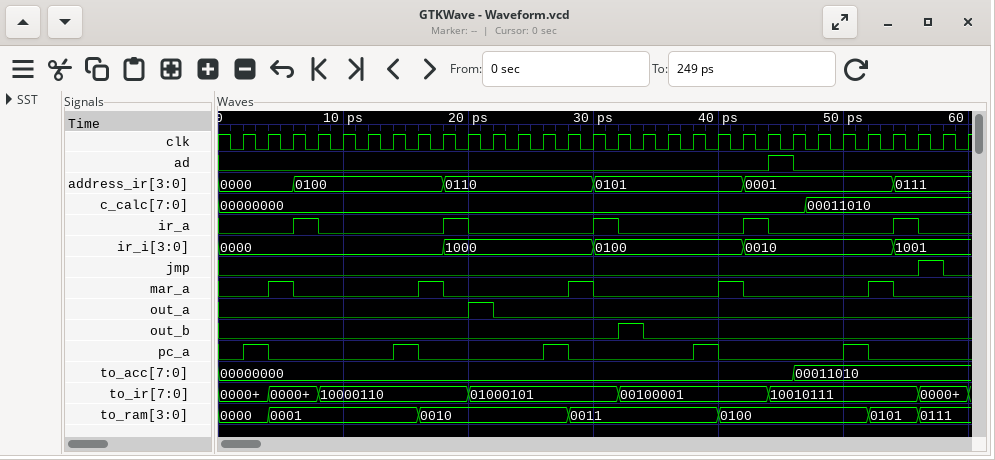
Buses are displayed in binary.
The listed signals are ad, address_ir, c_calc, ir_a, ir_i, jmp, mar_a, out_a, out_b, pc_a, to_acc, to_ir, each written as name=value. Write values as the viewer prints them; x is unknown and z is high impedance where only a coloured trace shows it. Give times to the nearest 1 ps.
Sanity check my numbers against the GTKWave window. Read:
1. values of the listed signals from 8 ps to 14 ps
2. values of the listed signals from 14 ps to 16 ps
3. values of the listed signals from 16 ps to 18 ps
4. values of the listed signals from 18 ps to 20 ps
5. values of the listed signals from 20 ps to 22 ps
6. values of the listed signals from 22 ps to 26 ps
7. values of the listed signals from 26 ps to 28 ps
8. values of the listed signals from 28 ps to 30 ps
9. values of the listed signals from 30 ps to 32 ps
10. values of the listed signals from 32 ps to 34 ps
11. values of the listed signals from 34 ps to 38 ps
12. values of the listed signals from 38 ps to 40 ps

ad=0, address_ir=0100, c_calc=00000000, ir_a=0, ir_i=0000, jmp=0, mar_a=0, out_a=0, out_b=0, pc_a=0, to_acc=00000000, to_ir=10000110
ad=0, address_ir=0100, c_calc=00000000, ir_a=0, ir_i=0000, jmp=0, mar_a=0, out_a=0, out_b=0, pc_a=1, to_acc=00000000, to_ir=10000110
ad=0, address_ir=0100, c_calc=00000000, ir_a=0, ir_i=0000, jmp=0, mar_a=1, out_a=0, out_b=0, pc_a=0, to_acc=00000000, to_ir=10000110
ad=0, address_ir=0110, c_calc=00000000, ir_a=1, ir_i=1000, jmp=0, mar_a=0, out_a=0, out_b=0, pc_a=0, to_acc=00000000, to_ir=10000110
ad=0, address_ir=0110, c_calc=00000000, ir_a=0, ir_i=1000, jmp=0, mar_a=0, out_a=1, out_b=0, pc_a=0, to_acc=00000000, to_ir=01000101
ad=0, address_ir=0110, c_calc=00000000, ir_a=0, ir_i=1000, jmp=0, mar_a=0, out_a=0, out_b=0, pc_a=0, to_acc=00000000, to_ir=01000101
ad=0, address_ir=0110, c_calc=00000000, ir_a=0, ir_i=1000, jmp=0, mar_a=0, out_a=0, out_b=0, pc_a=1, to_acc=00000000, to_ir=01000101
ad=0, address_ir=0110, c_calc=00000000, ir_a=0, ir_i=1000, jmp=0, mar_a=1, out_a=0, out_b=0, pc_a=0, to_acc=00000000, to_ir=01000101
ad=0, address_ir=0101, c_calc=00000000, ir_a=1, ir_i=0100, jmp=0, mar_a=0, out_a=0, out_b=0, pc_a=0, to_acc=00000000, to_ir=01000101
ad=0, address_ir=0101, c_calc=00000000, ir_a=0, ir_i=0100, jmp=0, mar_a=0, out_a=0, out_b=1, pc_a=0, to_acc=00000000, to_ir=00100001
ad=0, address_ir=0101, c_calc=00000000, ir_a=0, ir_i=0100, jmp=0, mar_a=0, out_a=0, out_b=0, pc_a=0, to_acc=00000000, to_ir=00100001
ad=0, address_ir=0101, c_calc=00000000, ir_a=0, ir_i=0100, jmp=0, mar_a=0, out_a=0, out_b=0, pc_a=1, to_acc=00000000, to_ir=00100001
